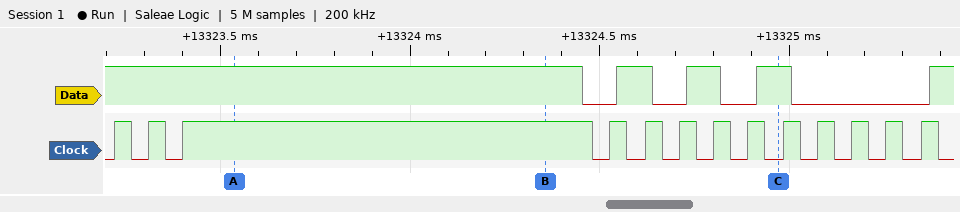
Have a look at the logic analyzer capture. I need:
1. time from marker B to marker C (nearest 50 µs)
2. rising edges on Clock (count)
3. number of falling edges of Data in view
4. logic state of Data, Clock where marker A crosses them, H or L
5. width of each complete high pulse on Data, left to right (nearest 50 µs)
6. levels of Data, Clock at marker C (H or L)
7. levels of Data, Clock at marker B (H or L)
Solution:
600 µs
13
4
Data=H, Clock=H
100 µs, 100 µs, 100 µs
Data=H, Clock=L
Data=H, Clock=H
